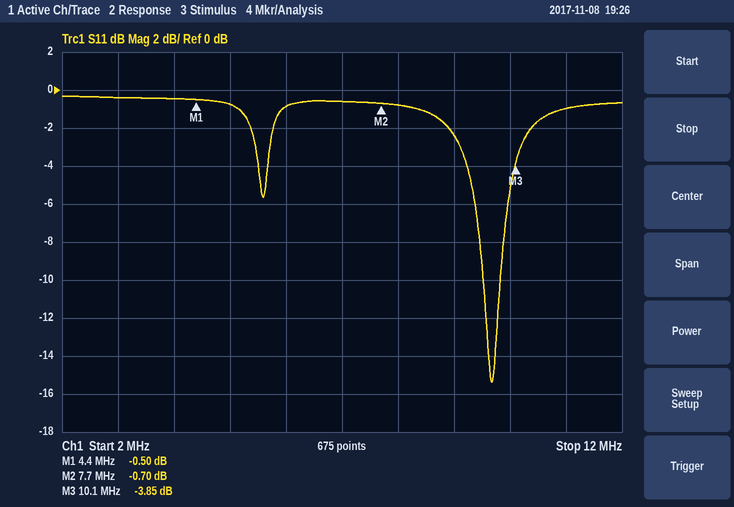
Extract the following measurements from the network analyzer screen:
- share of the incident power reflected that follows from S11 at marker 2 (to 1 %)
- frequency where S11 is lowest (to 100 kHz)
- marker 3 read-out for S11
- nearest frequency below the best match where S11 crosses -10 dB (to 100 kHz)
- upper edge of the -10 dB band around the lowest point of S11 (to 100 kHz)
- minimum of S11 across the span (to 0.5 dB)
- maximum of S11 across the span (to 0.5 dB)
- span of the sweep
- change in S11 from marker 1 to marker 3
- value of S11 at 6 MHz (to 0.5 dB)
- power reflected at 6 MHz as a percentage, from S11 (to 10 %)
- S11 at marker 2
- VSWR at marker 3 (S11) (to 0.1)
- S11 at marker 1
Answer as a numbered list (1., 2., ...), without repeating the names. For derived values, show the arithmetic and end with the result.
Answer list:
1. 10^(-0.7/10) ≈ 85 %
2. 9.7 MHz
3. -3.85 dB
4. 9.5 MHz
5. 9.8 MHz
6. -15.5 dB
7. -0.5 dB
8. 10 MHz
9. -3.85 − (-0.5) = -3.35 dB
10. -1.0 dB
11. 10^(-1/10) ≈ 79.4 %, so 80 % to the nearest 10 %
12. -0.70 dB
13. (1 + 0.6419)/(1 − 0.6419) ≈ 4.6
14. -0.50 dB
